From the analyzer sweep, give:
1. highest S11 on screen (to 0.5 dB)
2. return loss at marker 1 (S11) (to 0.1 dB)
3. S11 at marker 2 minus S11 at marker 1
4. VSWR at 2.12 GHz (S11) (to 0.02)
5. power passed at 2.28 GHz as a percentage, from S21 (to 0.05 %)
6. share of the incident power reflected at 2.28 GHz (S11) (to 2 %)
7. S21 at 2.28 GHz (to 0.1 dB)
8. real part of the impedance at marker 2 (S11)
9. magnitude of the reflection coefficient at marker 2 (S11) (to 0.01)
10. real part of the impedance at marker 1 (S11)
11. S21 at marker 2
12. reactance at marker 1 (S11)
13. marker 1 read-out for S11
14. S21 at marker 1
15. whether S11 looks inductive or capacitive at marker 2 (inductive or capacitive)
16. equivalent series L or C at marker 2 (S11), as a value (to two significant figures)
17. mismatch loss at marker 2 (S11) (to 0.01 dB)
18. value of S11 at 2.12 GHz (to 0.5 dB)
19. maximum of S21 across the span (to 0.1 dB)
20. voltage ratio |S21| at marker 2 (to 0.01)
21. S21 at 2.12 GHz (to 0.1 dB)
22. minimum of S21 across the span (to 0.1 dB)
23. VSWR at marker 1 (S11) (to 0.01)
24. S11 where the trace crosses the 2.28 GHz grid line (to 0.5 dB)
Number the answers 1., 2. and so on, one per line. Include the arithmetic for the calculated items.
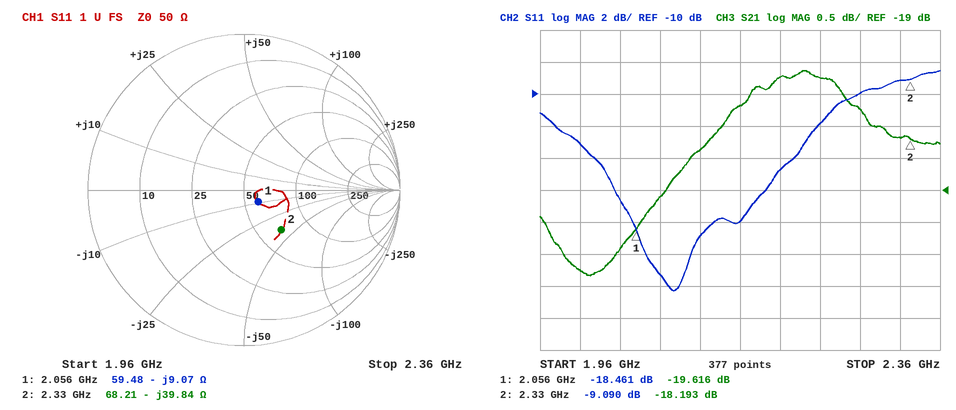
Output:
1. -8.5 dB
2. 18.5 dB
3. -9.09 − (-18.461) = 9.371 dB
4. |Γ| = 10^(-19/20) = 0.1122; VSWR = (1 + 0.1122)/(1 − 0.1122) ≈ 1.25, so 1.26 to the nearest 0.02
5. 10^(-17.7/10) ≈ 1.70 %
6. 10^(-10/10) ≈ 10 %
7. -17.7 dB
8. 68.21 Ω
9. 0.35
10. 59.48 Ω
11. -18.193 dB
12. -9.07 Ω
13. -18.461 dB
14. -19.616 dB
15. capacitive
16. C = 1/(2π × 2.33 GHz × 39.84 Ω) ≈ 1.7 pF
17. −10 log10(1 − 10^(-9.09/10)) ≈ 0.57 dB
18. -19.0 dB
19. -17.1 dB
20. 10^(-18.193/20) ≈ 0.12
21. -18.4 dB
22. -20.3 dB
23. (1 + 0.1194)/(1 − 0.1194) ≈ 1.27
24. -10.0 dB
